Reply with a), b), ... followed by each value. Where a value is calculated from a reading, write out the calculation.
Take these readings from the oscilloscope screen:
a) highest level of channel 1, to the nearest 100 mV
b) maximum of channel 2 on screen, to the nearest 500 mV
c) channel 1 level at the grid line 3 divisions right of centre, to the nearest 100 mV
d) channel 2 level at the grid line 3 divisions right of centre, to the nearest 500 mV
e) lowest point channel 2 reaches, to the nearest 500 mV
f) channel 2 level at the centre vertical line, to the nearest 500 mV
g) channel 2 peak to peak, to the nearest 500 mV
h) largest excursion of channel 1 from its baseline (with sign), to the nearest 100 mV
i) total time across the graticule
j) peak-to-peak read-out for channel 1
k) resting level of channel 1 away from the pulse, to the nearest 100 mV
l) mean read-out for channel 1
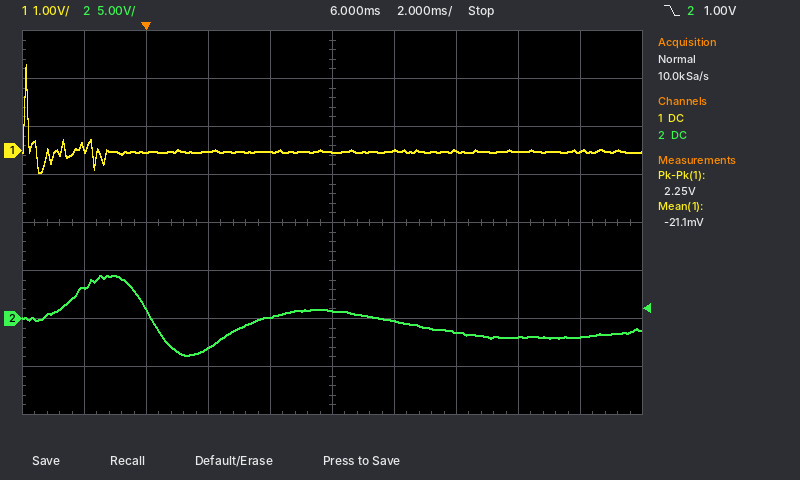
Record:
a) 1.8 V
b) 4.5 V
c) 0.0 V
d) -2.0 V
e) -4.0 V
f) 1.0 V
g) 4.5 V − (-4.0 V) = 8.5 V
h) 1.8 V − (0.0 V) = +1.8 V
i) 20 ms
j) 2.25 V
k) 0.0 V
l) -21.1 mV
